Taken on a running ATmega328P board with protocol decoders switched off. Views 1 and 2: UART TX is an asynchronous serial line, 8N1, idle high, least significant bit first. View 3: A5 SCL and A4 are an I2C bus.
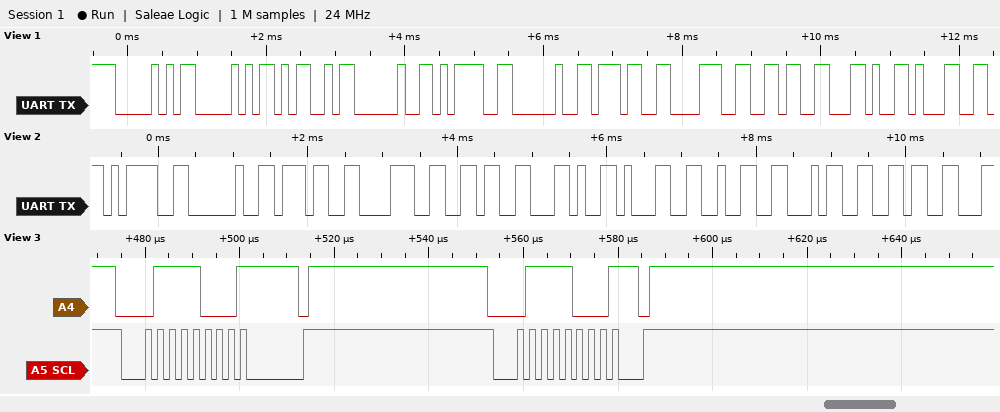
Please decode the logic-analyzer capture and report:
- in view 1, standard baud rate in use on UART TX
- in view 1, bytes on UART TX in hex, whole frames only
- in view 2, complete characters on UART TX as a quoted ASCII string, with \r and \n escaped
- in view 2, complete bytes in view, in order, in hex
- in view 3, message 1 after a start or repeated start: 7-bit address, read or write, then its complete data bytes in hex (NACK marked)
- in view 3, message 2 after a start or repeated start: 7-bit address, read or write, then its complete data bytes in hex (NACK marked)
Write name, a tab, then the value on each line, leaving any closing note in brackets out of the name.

in view 1, standard baud rate in use on UART TX	9600 baud
in view 1, bytes on UART TX in hex, whole frames only	50 50 4D 20 3D 20 37 38 36 2C 31
in view 2, complete characters on UART TX as a quoted ASCII string, with \r and \n escaped	"= 786,1246"
in view 2, complete bytes in view, in order, in hex	3D 20 37 38 36 2C 31 32 34 36
in view 3, message 1 after a start or repeated start: 7-bit address, read or write, then its complete data bytes in hex	0x3C write NACK
in view 3, message 2 after a start or repeated start: 7-bit address, read or write, then its complete data bytes in hex	0x3C write NACK
